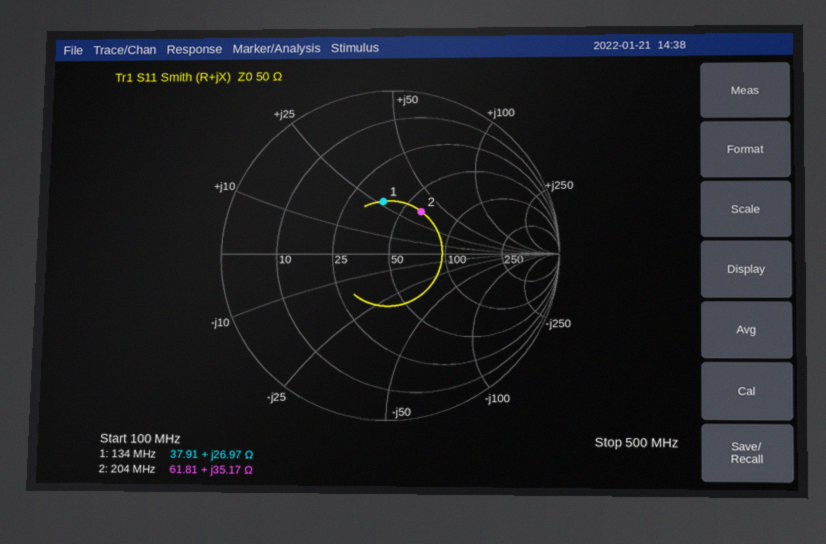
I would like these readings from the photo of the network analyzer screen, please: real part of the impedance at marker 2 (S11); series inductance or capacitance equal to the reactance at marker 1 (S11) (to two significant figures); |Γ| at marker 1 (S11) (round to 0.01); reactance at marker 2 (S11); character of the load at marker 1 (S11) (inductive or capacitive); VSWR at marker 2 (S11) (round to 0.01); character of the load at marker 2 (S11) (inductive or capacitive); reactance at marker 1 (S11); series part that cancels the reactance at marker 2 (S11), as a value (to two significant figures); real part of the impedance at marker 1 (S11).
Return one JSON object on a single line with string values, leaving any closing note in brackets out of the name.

{"real part of the impedance at marker 2": "61.81 Ω", "series inductance or capacitance equal to the reactance at marker 1 (S11)": "32 nH", "|Γ| at marker 1 (S11)": "0.32", "reactance at marker 2": "+35.17 Ω", "character of the load at marker 1 (S11)": "inductive", "VSWR at marker 2 (S11)": "1.93", "character of the load at marker 2 (S11)": "inductive", "reactance at marker 1": "+26.97 Ω", "series part that cancels the reactance at marker 2 (S11), as a value": "22 pF", "real part of the impedance at marker 1": "37.91 Ω"}
